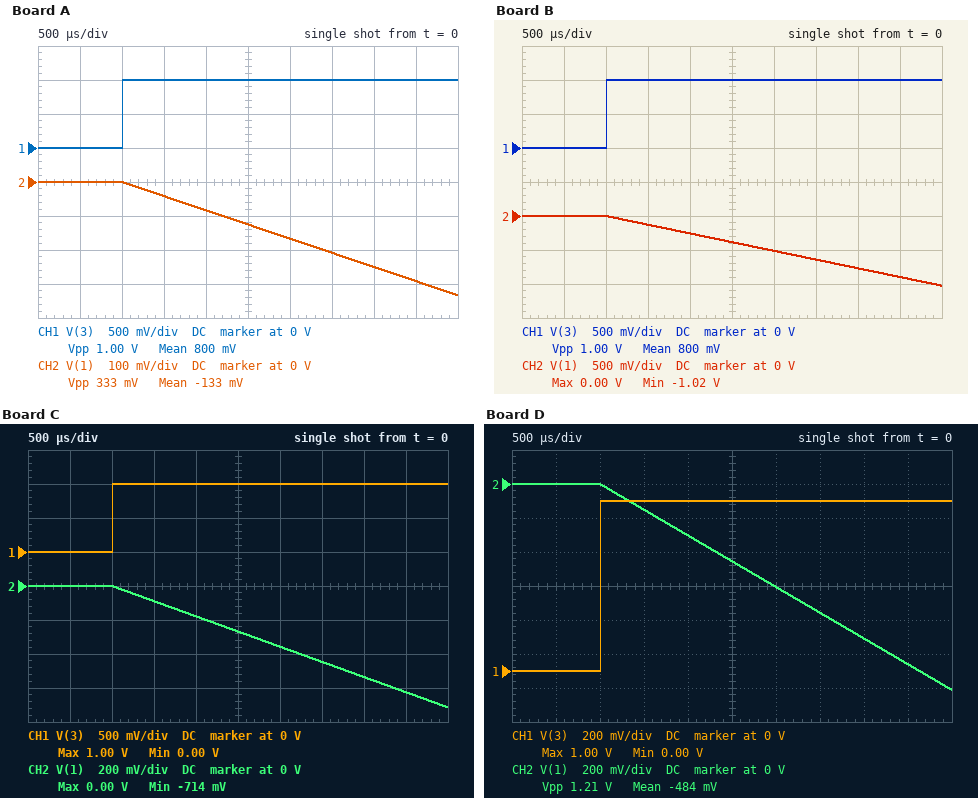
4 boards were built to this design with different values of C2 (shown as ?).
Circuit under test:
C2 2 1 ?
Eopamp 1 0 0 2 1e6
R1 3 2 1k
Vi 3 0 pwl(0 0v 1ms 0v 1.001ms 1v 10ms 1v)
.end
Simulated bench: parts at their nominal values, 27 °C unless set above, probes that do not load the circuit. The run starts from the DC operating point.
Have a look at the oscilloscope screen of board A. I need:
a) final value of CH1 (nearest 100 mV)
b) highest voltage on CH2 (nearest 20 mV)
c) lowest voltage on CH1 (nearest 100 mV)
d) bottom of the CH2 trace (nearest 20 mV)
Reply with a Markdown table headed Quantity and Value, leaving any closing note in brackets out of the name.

| Quantity | Value |
|---|---|
| final value of CH1 | 1.0 V |
| highest voltage on CH2 | 0 V |
| lowest voltage on CH1 | 0 V |
| bottom of the CH2 trace | -340 mV |
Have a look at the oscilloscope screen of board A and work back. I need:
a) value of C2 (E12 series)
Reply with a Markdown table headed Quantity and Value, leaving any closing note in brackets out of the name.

| Quantity | Value |
|---|---|
| value of C2 | 12 µF |
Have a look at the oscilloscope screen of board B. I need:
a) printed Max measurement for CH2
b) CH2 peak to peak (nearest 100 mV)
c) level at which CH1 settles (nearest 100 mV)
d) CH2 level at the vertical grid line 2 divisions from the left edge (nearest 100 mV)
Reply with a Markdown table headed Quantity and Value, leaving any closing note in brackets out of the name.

| Quantity | Value |
|---|---|
| printed Max measurement for CH2 | 0.00 V |
| CH2 peak to peak | 1.0 V |
| level at which CH1 settles | 1.0 V |
| CH2 level at the vertical grid line 2 divisions from the left edge | 0 V |
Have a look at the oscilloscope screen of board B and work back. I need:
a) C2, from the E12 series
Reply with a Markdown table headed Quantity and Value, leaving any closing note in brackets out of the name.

| Quantity | Value |
|---|---|
| C2, from the E12 series | 3.9 µF |
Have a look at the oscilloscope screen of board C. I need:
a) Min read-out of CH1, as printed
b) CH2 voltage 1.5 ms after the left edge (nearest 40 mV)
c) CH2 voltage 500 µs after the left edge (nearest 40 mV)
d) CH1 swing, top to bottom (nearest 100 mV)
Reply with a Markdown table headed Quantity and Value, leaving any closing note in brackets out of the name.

| Quantity | Value |
|---|---|
| Min read-out of CH1, as printed | 0.00 V |
| CH2 voltage 1.5 ms after the left edge | -80 mV |
| CH2 voltage 500 µs after the left edge | 0 V |
| CH1 swing, top to bottom | 1.0 V |
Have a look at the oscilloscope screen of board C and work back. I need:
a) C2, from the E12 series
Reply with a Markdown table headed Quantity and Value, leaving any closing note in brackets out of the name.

| Quantity | Value |
|---|---|
| C2, from the E12 series | 5.6 µF |
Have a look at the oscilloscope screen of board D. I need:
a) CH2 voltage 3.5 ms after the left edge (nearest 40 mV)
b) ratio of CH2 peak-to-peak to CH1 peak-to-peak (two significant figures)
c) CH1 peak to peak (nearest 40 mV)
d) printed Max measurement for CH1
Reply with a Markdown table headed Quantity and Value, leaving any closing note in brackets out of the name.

| Quantity | Value |
|---|---|
| CH2 voltage 3.5 ms after the left edge | -760 mV |
| ratio of CH2 peak-to-peak to CH1 peak-to-peak | 1.2 |
| CH1 peak to peak | 1.00 V |
| printed Max measurement for CH1 | 1.00 V |
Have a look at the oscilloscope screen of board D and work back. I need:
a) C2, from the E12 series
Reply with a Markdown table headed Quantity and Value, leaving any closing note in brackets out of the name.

| Quantity | Value |
|---|---|
| C2, from the E12 series | 3.3 µF |
